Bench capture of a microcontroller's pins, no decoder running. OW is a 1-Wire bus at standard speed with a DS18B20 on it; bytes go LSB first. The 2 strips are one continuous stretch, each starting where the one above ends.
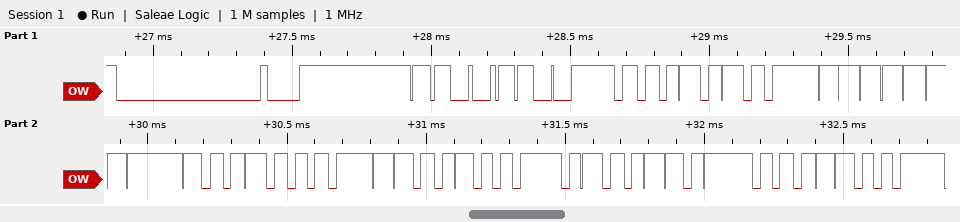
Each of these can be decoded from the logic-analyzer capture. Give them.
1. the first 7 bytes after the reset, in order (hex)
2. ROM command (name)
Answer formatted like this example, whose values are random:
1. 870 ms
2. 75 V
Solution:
1. 33 28 FF 09 13 B2 18
2. Read ROM
